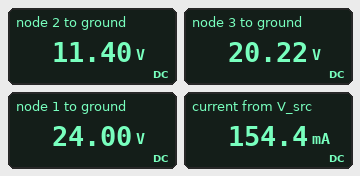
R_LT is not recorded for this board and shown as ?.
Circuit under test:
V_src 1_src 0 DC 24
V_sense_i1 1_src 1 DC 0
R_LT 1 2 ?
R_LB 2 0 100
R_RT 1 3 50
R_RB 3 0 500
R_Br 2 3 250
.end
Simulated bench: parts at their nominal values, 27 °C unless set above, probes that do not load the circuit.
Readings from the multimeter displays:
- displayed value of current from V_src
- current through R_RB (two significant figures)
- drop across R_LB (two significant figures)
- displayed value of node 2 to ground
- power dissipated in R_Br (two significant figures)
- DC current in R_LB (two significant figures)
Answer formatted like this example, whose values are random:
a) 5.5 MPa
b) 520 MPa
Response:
a) 154.4 mA
b) 40 mA
c) 11 V
d) 11.40 V
e) 310 mW
f) 110 mA
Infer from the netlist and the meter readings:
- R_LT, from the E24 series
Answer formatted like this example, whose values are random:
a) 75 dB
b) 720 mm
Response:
a) 160 Ω
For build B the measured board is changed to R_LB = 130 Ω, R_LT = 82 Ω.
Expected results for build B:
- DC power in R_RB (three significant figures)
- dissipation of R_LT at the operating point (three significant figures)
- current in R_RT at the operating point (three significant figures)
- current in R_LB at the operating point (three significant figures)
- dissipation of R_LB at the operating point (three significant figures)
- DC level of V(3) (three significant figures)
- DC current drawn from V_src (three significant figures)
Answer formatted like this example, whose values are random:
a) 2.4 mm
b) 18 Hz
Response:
a) 872 mW
b) 830 mW
c) 62.3 mA
d) 121 mA
e) 1.91 W
f) 20.9 V
g) 163 mA
